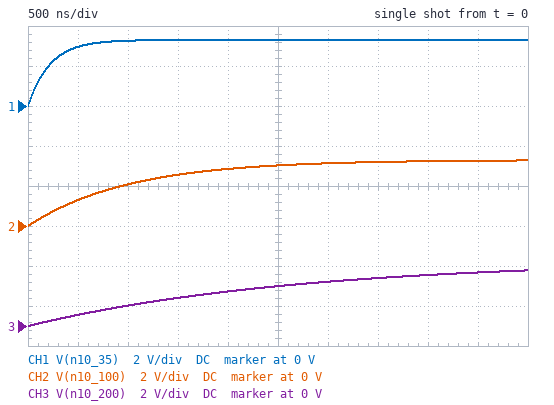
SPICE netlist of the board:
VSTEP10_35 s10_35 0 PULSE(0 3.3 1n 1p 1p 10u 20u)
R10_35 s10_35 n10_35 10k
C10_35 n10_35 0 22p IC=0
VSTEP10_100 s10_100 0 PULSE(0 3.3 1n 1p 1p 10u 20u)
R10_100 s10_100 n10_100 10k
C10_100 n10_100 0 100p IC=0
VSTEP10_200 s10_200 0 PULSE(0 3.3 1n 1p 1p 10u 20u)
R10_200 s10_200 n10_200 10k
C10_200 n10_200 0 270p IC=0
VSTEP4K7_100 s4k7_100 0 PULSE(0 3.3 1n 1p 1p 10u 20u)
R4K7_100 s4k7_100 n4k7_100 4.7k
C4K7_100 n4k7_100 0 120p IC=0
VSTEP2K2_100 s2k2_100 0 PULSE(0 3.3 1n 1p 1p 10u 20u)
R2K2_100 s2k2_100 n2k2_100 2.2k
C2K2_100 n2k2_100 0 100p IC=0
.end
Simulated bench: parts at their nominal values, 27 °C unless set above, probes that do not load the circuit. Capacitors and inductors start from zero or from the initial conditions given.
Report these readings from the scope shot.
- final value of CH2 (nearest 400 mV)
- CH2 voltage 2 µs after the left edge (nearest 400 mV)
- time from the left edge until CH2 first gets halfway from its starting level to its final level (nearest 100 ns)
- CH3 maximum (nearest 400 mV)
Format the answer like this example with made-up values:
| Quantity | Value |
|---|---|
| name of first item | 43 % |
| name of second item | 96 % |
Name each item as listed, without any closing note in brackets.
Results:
| Quantity | Value |
|---|---|
| final value of CH2 | 3.2 V |
| CH2 voltage 2 µs after the left edge | 2.8 V |
| time from the left edge until CH2 first gets halfway from its starting level to its final level | 700 ns |
| CH3 maximum | 2.8 V |
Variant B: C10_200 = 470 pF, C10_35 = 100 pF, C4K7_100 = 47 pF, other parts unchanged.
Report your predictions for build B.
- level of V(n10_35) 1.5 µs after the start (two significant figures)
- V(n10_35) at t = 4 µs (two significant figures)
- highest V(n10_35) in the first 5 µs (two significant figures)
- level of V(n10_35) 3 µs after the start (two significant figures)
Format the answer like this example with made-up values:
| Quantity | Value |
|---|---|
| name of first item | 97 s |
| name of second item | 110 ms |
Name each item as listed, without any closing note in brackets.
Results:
| Quantity | Value |
|---|---|
| level of V(n10_35) 1.5 µs after the start | 2.6 V |
| V(n10_35) at t = 4 µs | 3.2 V |
| highest V(n10_35) in the first 5 µs | 3.3 V |
| level of V(n10_35) 3 µs after the start | 3.1 V |
